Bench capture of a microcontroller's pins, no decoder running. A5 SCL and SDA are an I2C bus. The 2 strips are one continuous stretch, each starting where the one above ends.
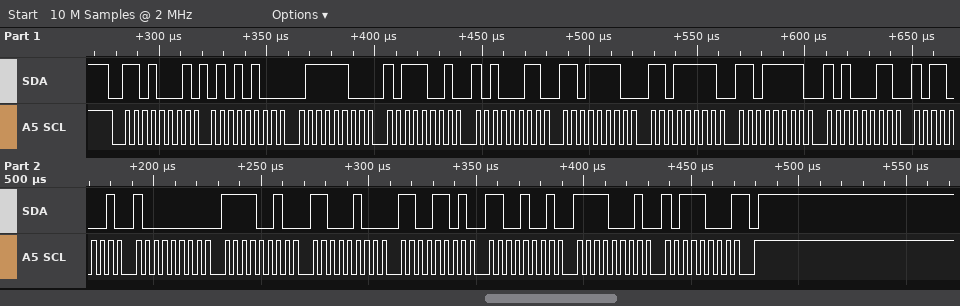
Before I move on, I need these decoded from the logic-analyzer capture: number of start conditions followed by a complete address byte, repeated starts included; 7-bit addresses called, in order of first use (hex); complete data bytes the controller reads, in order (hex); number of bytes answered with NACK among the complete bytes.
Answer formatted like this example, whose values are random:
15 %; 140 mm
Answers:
1; 0x68; 54 7C B9 A3 DE DF DF A3 B1 80 F2 C4 CD C9 F1 B8; 1
